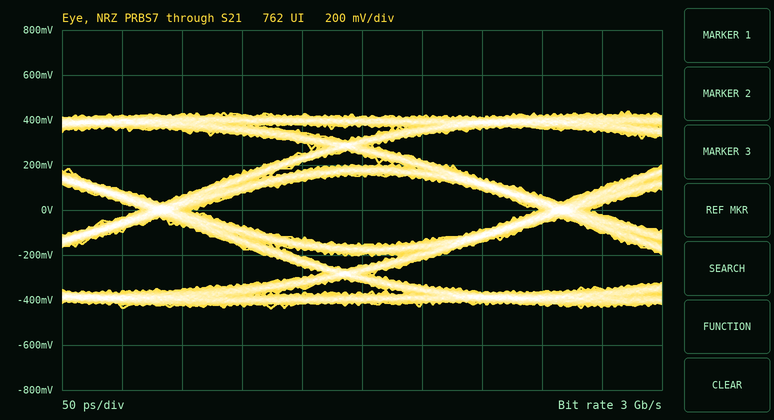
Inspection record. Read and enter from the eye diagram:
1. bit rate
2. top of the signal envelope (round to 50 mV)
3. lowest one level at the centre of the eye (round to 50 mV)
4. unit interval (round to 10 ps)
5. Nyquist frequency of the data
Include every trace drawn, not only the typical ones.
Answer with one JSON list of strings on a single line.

["3 Gb/s", "450 mV", "150 mV", "330 ps", "1.5 GHz"]
